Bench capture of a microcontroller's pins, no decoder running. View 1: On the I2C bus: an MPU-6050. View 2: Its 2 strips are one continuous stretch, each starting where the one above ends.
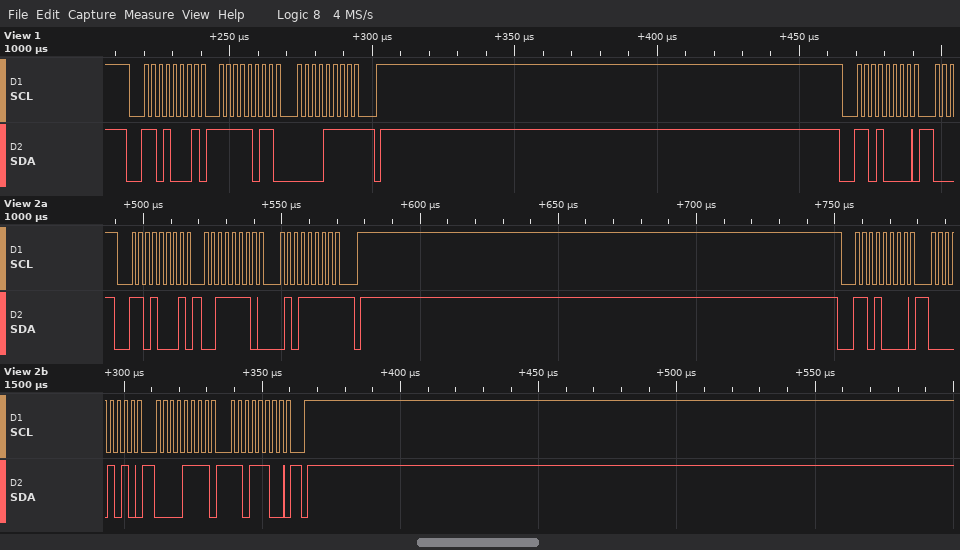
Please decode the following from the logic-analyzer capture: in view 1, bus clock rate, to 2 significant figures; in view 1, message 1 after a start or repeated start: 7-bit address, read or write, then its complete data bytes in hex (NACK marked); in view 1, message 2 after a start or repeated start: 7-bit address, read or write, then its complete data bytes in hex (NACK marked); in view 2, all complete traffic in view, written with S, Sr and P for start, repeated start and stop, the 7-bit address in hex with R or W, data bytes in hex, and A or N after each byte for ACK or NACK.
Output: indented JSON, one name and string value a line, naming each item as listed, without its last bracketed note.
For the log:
{
  "in view 1, bus clock rate, to 2 significant figures": "400 kHz",
  "in view 1, message 1 after a start or repeated start: 7-bit address, read or write, then its complete data bytes in hex": "0x68 read: FB 0F NACK",
  "in view 1, message 2 after a start or repeated start: 7-bit address, read or write, then its complete data bytes in hex": "0x68 write",
  "in view 2, all complete traffic in view, written with S, Sr and P for start, repeated start and stop, the 7-bit address in hex with R or W, data bytes in hex, and A or N after each byte for ACK or NACK": "S 68R A 3E A 5F N P S 68W A 0A A 0F A DC A P"
}
